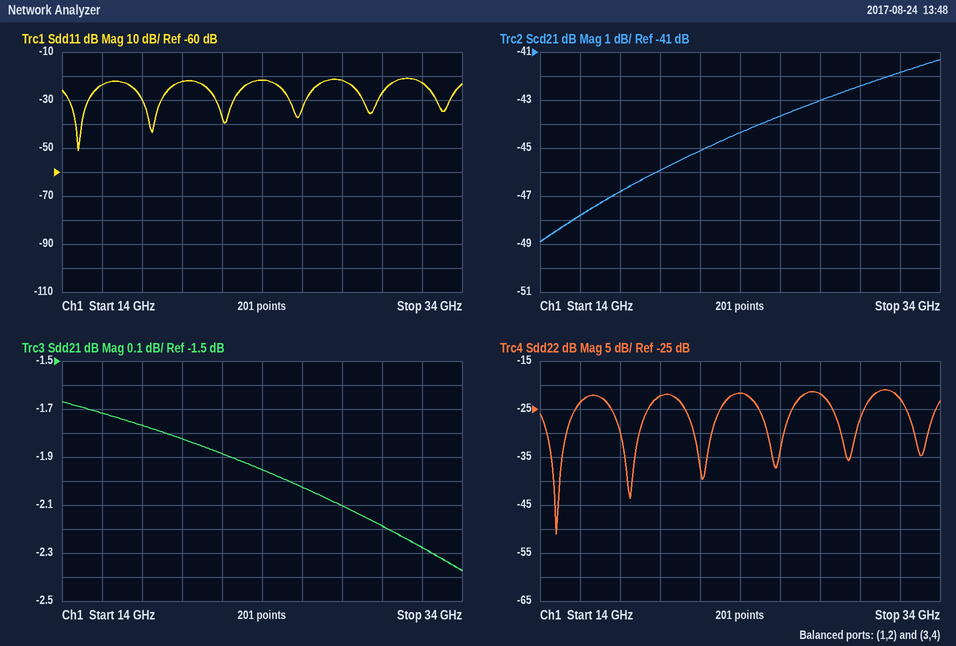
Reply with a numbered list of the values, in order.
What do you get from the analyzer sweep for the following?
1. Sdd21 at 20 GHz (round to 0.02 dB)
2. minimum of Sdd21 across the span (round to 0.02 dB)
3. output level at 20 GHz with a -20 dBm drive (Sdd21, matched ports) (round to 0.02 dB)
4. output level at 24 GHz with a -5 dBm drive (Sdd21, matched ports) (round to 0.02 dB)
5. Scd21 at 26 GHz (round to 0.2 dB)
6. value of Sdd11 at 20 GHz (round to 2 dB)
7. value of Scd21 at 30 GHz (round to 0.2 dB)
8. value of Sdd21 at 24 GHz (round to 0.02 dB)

1. -1.82 dB
2. -2.38 dB
3. -21.82 dBm
4. -6.96 dBm
5. -43.6 dB
6. -22 dB
7. -42.4 dB
8. -1.96 dB
